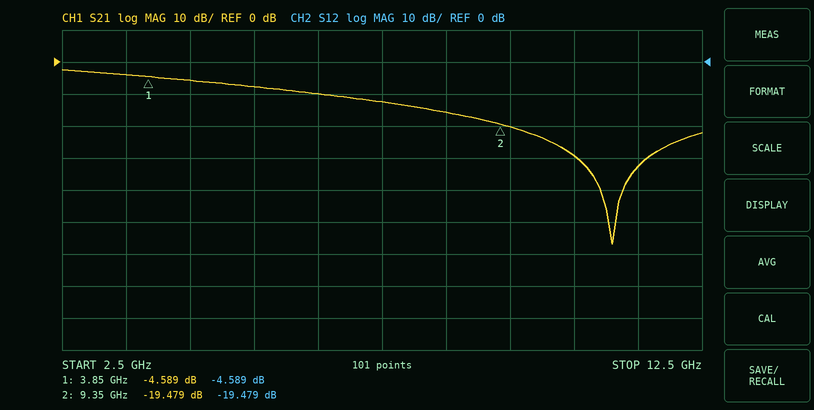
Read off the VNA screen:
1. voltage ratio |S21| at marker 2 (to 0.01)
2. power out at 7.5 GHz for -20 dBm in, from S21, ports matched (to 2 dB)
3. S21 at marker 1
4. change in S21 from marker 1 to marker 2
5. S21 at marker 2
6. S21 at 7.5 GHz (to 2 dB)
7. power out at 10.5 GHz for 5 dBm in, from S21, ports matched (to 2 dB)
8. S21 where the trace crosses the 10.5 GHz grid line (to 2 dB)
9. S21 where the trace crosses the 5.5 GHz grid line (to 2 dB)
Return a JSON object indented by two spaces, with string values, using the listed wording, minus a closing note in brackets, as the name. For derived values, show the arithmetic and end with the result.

{
  "voltage ratio |S21| at marker 2": "10^(-19.479/20) ≈ 0.11",
  "power out at 7.5 GHz for -20 dBm in, from S21, ports matched": "-20 dBm + (-12 dB) = -32 dBm",
  "S21 at marker 1": "-4.589 dB",
  "change in S21 from marker 1 to marker 2": "-19.479 − (-4.589) = -14.890 dB",
  "S21 at marker 2": "-19.479 dB",
  "S21 at 7.5 GHz": "-12 dB",
  "power out at 10.5 GHz for 5 dBm in, from S21, ports matched": "5 dBm + (-30 dB) = -24 dBm",
  "S21 where the trace crosses the 10.5 GHz grid line": "-30 dB",
  "S21 where the trace crosses the 5.5 GHz grid line": "-8 dB"
}
